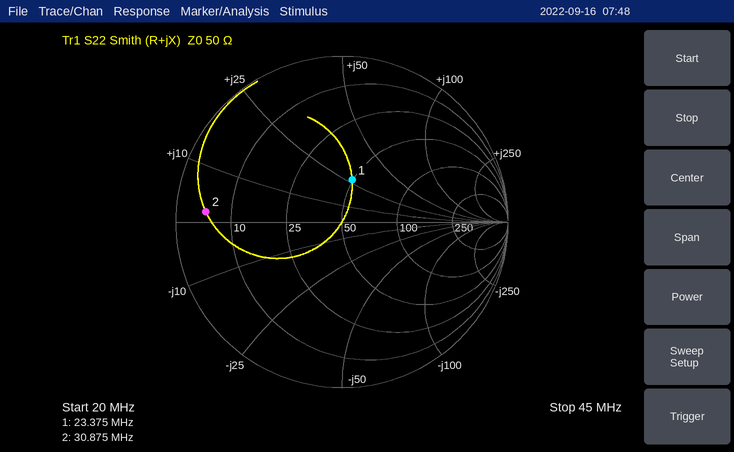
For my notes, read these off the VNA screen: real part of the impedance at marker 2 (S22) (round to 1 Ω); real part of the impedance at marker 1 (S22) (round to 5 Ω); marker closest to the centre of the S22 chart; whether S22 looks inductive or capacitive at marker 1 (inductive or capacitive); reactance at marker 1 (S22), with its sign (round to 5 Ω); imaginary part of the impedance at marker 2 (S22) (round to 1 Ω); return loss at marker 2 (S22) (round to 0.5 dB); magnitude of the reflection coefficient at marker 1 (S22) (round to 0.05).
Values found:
5 Ω
50 Ω
marker 1
inductive
+25 Ω
+2 Ω
1.5 dB
0.25
